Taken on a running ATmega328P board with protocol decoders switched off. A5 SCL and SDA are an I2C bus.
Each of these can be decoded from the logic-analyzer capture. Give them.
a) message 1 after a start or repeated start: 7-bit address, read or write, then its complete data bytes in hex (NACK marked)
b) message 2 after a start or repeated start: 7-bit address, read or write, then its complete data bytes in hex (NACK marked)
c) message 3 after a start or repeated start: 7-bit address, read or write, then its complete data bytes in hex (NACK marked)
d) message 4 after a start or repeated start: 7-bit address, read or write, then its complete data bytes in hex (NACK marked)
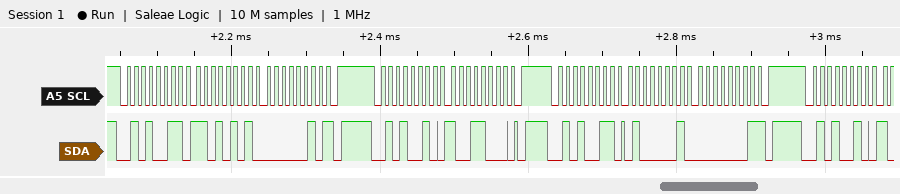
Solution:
0x29 read: D5 02 NACK
0x29 write: 98
0x29 read: 41 01 NACK
0x29 write
